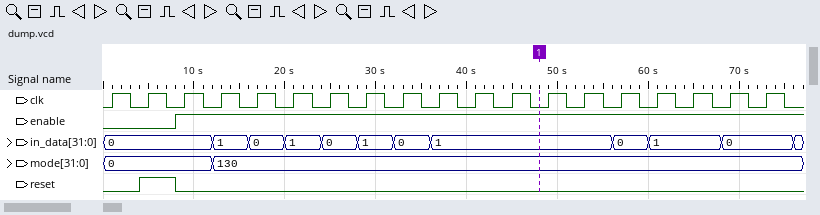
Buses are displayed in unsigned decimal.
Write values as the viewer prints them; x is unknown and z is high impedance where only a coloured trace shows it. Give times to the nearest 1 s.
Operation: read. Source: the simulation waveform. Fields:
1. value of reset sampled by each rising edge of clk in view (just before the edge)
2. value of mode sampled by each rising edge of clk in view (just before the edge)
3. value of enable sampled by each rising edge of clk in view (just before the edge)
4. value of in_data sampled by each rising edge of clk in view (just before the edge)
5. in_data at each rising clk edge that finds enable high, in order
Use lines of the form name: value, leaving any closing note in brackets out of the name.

value of reset sampled by each rising edge of clk in view: 0 1 0 0 0 0 0 0 0 0 0 0 0 0 0 0 0 0 0
value of mode sampled by each rising edge of clk in view: 0, 0, 0, 130, 130, 130, 130, 130, 130, 130, 130, 130, 130, 130, 130, 130, 130, 130, 130
value of enable sampled by each rising edge of clk in view: 0 0 1 1 1 1 1 1 1 1 1 1 1 1 1 1 1 1 1
value of in_data sampled by each rising edge of clk in view: 0, 0, 0, 1, 0, 1, 0, 1, 0, 1, 1, 1, 1, 1, 0, 1, 1, 0, 0
in_data at each rising clk edge that finds enable high, in order: 0, 1, 0, 1, 0, 1, 0, 1, 1, 1, 1, 1, 0, 1, 1, 0, 0
